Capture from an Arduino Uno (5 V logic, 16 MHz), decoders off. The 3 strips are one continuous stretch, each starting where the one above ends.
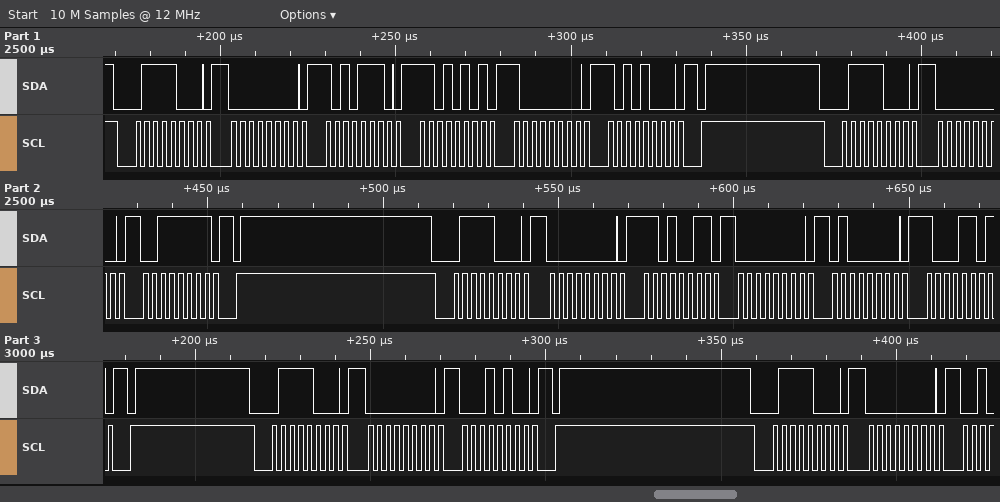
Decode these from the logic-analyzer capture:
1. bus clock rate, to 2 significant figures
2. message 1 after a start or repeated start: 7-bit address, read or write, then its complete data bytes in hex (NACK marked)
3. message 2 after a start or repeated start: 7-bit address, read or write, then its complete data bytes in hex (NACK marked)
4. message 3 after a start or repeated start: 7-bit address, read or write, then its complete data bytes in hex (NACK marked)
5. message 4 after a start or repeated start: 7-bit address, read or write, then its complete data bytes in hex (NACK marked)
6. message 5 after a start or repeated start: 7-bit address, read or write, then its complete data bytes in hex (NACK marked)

400 kHz
0x3C write: 00 AE D5 80 A8
0x3C write: 00 3F
0x3C write: 00 D3 00 40 8D
0x3C write: 00 14
0x3C write: 00
